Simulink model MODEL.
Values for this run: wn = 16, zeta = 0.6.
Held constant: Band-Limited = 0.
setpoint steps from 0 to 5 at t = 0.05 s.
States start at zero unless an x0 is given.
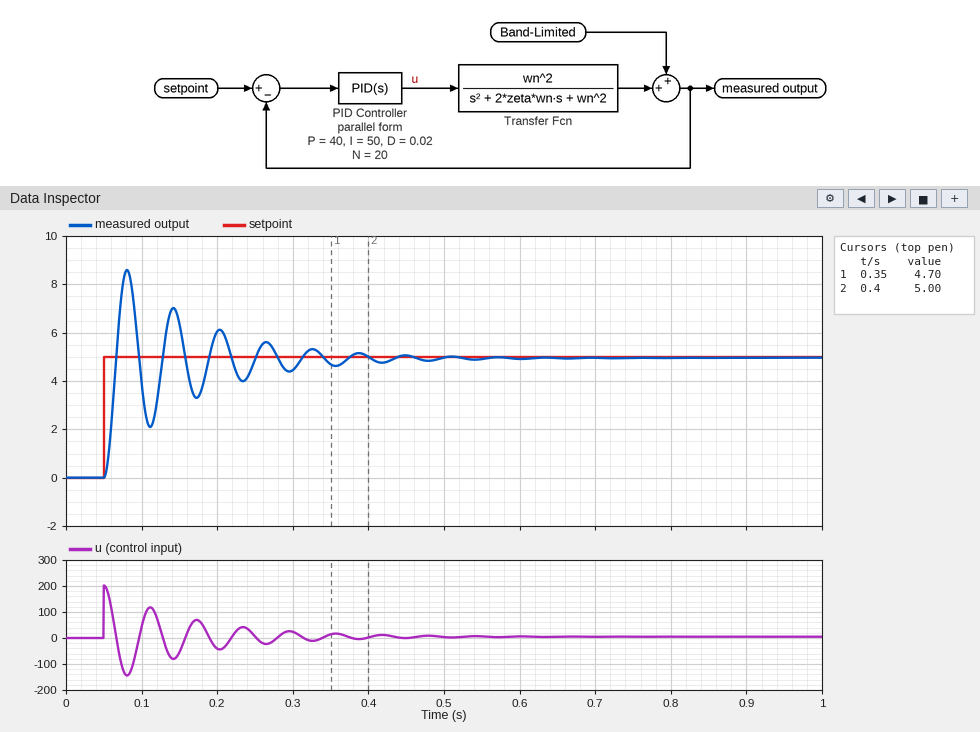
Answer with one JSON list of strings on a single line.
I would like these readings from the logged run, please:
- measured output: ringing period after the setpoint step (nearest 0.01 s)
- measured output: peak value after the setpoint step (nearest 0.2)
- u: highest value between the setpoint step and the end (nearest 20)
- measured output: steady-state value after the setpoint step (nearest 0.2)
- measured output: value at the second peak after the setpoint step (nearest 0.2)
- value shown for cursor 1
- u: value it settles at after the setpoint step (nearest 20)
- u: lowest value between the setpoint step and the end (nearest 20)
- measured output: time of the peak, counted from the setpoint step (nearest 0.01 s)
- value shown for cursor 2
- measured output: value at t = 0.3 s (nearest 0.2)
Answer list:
["0.06 s", "8.6", "200", "5.0", "7.0", "4.70", "0", "-140", "0.03 s", "5.00", "4.4"]
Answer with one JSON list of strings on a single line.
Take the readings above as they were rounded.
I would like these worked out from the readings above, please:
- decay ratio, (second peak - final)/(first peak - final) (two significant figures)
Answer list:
["0.56"]
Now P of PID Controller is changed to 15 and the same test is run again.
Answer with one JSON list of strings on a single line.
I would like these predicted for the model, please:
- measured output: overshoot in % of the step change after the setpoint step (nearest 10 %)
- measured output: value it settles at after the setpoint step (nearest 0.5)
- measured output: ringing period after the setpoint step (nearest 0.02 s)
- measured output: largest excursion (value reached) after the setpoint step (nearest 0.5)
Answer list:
["60 %", "5.0", "0.10 s", "8.0"]
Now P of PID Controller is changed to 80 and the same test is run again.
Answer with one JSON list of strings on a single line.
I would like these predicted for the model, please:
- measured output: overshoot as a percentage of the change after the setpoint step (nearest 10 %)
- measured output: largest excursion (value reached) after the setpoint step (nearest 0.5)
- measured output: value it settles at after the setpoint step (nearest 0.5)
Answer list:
["80 %", "9.0", "5.0"]
